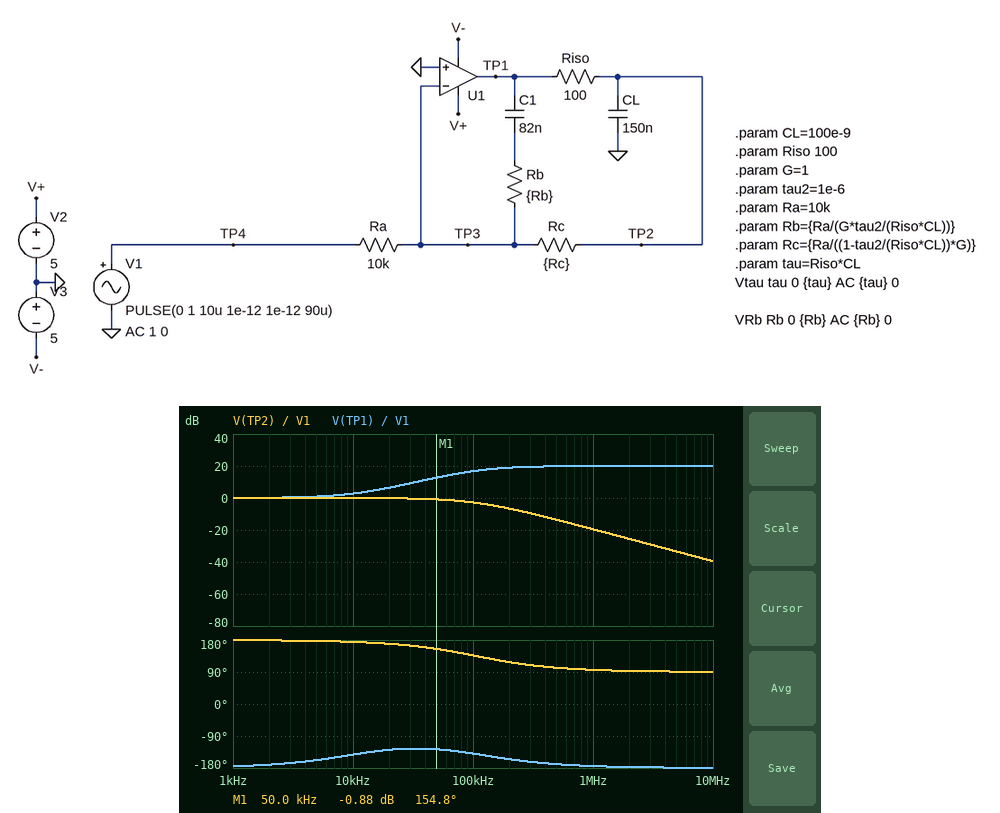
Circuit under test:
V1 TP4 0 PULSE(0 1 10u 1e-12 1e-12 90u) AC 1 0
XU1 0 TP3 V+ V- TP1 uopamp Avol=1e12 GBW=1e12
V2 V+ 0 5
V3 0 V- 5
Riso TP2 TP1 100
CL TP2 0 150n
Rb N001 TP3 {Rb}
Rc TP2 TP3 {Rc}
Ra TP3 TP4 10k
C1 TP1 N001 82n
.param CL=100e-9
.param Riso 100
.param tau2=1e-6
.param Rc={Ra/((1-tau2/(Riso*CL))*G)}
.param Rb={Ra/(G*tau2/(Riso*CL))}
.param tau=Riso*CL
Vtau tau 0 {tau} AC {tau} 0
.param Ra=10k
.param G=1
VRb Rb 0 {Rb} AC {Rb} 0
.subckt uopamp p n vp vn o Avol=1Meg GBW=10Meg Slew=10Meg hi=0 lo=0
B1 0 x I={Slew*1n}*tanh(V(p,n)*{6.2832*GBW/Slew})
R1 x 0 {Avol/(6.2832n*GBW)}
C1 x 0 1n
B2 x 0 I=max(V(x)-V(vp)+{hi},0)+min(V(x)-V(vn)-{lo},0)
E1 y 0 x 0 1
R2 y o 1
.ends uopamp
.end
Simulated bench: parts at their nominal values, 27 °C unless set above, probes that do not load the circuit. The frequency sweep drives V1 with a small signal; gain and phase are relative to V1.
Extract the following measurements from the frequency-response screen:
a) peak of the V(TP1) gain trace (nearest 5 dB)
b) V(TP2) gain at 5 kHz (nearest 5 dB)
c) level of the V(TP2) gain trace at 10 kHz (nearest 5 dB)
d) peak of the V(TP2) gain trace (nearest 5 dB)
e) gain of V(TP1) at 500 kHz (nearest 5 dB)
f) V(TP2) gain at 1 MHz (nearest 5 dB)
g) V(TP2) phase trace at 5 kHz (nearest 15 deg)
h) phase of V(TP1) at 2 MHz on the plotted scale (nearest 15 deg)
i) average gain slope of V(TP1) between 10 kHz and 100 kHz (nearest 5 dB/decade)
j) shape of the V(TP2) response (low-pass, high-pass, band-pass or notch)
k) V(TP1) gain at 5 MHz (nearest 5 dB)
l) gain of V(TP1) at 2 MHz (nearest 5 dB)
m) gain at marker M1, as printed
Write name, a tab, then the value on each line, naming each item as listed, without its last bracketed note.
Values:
peak of the V(TP1) gain trace	20 dB
V(TP2) gain at 5 kHz	0 dB
level of the V(TP2) gain trace at 10 kHz	0 dB
peak of the V(TP2) gain trace	0 dB
gain of V(TP1) at 500 kHz	20 dB
V(TP2) gain at 1 MHz	-20 dB
V(TP2) phase trace at 5 kHz	180 deg
phase of V(TP1) at 2 MHz on the plotted scale	-180 deg
average gain slope of V(TP1) between 10 kHz and 100 kHz	15 dB/decade
shape of the V(TP2) response	low-pass
V(TP1) gain at 5 MHz	20 dB
gain of V(TP1) at 2 MHz	20 dB
gain at marker M1, as printed	-0.88 dB
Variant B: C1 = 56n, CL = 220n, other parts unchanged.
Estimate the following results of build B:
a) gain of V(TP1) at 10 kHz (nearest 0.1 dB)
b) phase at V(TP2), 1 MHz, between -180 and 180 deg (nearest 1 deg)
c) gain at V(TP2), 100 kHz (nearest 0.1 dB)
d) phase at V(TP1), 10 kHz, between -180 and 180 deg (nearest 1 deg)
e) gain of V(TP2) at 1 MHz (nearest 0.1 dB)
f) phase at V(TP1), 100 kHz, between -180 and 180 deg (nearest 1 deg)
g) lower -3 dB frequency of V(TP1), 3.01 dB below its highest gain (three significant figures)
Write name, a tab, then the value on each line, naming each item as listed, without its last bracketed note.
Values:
gain of V(TP1) at 10 kHz	4.6 dB
phase at V(TP2), 1 MHz, between -180 and 180 deg	94 deg
gain at V(TP2), 100 kHz	-4.6 dB
phase at V(TP1), 10 kHz, between -180 and 180 deg	-134 deg
gain of V(TP2) at 1 MHz	-22.8 dB
phase at V(TP1), 100 kHz, between -180 and 180 deg	-148 deg
lower -3 dB frequency of V(TP1), 3.01 dB below its highest gain	71.6 kHz
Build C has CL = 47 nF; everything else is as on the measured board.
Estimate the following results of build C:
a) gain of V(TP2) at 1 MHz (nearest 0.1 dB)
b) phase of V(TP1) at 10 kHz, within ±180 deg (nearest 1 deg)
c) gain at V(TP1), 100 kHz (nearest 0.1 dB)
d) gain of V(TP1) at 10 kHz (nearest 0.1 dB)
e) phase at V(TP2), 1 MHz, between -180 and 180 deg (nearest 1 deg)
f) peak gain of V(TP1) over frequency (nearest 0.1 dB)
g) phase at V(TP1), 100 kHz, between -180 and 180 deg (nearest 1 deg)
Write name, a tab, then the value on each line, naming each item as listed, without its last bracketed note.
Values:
gain of V(TP2) at 1 MHz	-9.9 dB
phase of V(TP1) at 10 kHz, within ±180 deg	-165 deg
gain at V(TP1), 100 kHz	9.5 dB
gain of V(TP1) at 10 kHz	0.4 dB
phase at V(TP2), 1 MHz, between -180 and 180 deg	109 deg
peak gain of V(TP1) over frequency	20.0 dB
phase at V(TP1), 100 kHz, between -180 and 180 deg	-125 deg
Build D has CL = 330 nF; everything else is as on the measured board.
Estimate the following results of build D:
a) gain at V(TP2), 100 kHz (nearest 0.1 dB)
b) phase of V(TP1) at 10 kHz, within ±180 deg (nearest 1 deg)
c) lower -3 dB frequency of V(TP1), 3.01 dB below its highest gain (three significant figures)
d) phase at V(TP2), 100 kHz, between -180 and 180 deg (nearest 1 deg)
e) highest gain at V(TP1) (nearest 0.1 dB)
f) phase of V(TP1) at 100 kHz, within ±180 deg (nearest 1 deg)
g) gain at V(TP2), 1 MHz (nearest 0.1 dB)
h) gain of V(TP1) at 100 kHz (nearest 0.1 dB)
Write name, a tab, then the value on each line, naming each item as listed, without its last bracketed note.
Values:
gain at V(TP2), 100 kHz	-7.2 dB
phase of V(TP1) at 10 kHz, within ±180 deg	-128 deg
lower -3 dB frequency of V(TP1), 3.01 dB below its highest gain	47.8 kHz
phase at V(TP2), 100 kHz, between -180 and 180 deg	116 deg
highest gain at V(TP1)	20.0 dB
phase of V(TP1) at 100 kHz, within ±180 deg	-157 deg
gain at V(TP2), 1 MHz	-26.3 dB
gain of V(TP1) at 100 kHz	19.1 dB
